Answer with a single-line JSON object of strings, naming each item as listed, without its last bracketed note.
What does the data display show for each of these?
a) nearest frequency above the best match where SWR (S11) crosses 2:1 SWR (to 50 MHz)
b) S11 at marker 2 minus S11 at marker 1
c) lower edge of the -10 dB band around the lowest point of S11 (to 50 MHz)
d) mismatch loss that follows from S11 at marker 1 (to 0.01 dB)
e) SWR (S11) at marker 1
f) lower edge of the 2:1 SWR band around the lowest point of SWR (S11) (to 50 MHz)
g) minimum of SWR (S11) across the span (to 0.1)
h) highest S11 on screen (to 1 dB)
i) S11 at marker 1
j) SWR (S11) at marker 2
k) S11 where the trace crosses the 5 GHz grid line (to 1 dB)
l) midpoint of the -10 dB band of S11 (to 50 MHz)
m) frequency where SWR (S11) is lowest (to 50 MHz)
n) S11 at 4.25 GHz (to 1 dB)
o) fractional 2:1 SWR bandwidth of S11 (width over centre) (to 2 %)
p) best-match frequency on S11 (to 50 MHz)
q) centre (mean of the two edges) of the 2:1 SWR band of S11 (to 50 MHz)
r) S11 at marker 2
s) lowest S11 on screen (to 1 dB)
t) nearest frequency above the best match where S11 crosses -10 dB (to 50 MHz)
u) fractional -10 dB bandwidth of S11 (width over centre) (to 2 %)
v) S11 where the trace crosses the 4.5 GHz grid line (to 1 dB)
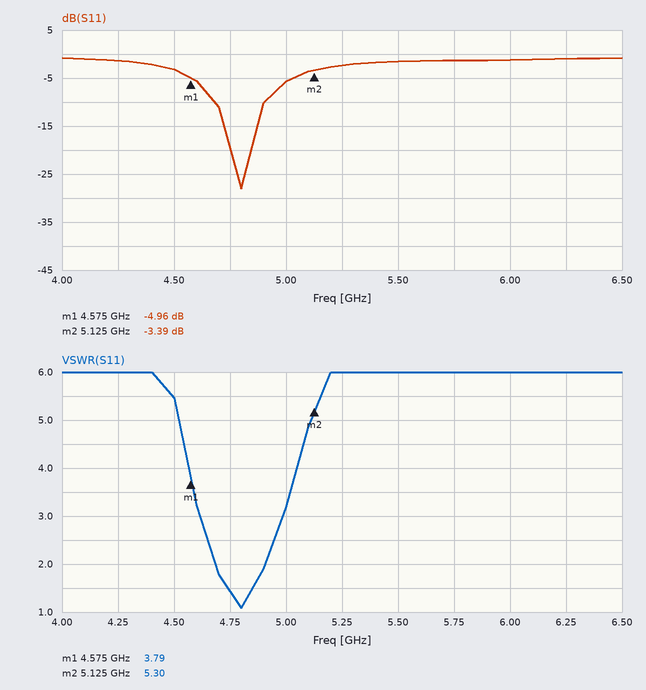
{"nearest frequency above the best match where SWR (S11) crosses 2:1 SWR": "4.90 GHz", "S11 at marker 2 minus S11 at marker 1": "1.57 dB", "lower edge of the -10 dB band around the lowest point of S11": "4.70 GHz", "mismatch loss that follows from S11 at marker 1": "1.67 dB", "SWR (S11) at marker 1": "3.79", "lower edge of the 2:1 SWR band around the lowest point of SWR (S11)": "4.70 GHz", "minimum of SWR (S11) across the span": "1.1", "highest S11 on screen": "-1 dB", "S11 at marker 1": "-4.96 dB", "SWR (S11) at marker 2": "5.30", "S11 where the trace crosses the 5 GHz grid line": "-6 dB", "midpoint of the -10 dB band of S11": "4.80 GHz", "frequency where SWR (S11) is lowest": "4.80 GHz", "S11 at 4.25 GHz": "-1 dB", "fractional 2:1 SWR bandwidth of S11 (width over centre)": "4 %", "best-match frequency on S11": "4.80 GHz", "centre (mean of the two edges) of the 2:1 SWR band of S11": "4.80 GHz", "S11 at marker 2": "-3.39 dB", "lowest S11 on screen": "-28 dB", "nearest frequency above the best match where S11 crosses -10 dB": "4.90 GHz", "fractional -10 dB bandwidth of S11 (width over centre)": "4 %", "S11 where the trace crosses the 4.5 GHz grid line": "-3 dB"}
